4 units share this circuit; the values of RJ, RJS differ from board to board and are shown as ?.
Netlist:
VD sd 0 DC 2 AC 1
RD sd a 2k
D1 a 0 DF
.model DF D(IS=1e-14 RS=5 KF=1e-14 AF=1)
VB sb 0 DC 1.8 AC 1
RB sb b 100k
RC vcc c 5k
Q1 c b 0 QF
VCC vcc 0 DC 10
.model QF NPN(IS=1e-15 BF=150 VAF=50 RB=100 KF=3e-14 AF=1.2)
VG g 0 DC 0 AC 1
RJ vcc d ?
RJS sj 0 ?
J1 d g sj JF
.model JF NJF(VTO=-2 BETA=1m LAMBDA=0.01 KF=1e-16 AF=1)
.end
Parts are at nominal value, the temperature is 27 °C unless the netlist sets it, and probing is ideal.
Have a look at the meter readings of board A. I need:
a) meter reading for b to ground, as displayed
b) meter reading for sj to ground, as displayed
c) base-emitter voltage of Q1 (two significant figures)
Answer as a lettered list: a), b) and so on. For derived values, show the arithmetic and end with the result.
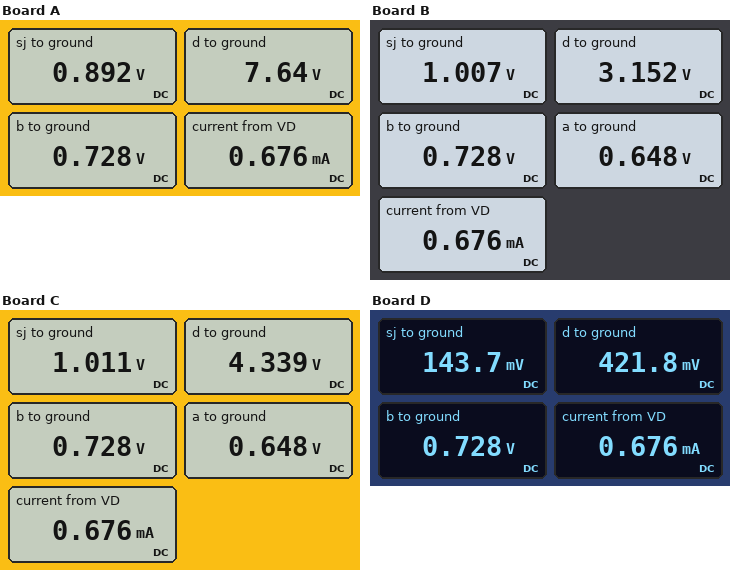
a) 0.728 V
b) 0.892 V
c) 728 mV = 730 mV
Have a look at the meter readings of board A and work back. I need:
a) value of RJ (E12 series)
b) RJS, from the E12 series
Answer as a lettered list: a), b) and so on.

a) 1.8 kΩ
b) 680 Ω
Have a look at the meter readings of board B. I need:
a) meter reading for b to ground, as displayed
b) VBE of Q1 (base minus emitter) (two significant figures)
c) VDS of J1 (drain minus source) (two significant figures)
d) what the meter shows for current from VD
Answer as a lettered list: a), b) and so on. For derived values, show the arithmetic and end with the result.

a) 0.728 V
b) 728 mV = 730 mV
c) 3.152 V - 1.007 V = 2.1 V
d) 0.676 mA
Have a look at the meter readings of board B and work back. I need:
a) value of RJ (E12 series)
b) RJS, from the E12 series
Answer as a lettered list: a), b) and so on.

a) 6.8 kΩ
b) 1 kΩ
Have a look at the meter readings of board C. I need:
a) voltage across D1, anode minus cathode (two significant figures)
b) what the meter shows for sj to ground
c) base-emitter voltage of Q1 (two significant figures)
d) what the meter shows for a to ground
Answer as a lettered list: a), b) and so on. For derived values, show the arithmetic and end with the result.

a) 648 mV = 650 mV
b) 1.011 V
c) 728 mV = 730 mV
d) 0.648 V
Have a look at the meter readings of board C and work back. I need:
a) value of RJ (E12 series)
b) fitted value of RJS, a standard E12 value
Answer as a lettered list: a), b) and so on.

a) 5.6 kΩ
b) 1 kΩ
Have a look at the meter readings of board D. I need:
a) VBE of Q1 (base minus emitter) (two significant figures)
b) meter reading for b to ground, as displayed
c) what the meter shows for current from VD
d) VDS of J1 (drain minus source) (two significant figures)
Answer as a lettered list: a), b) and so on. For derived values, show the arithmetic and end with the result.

a) 728 mV = 730 mV
b) 0.728 V
c) 0.676 mA
d) 421.8 mV - 143.7 mV = 280 mV
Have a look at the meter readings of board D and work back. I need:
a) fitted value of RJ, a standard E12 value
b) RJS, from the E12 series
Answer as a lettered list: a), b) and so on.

a) 10 kΩ
b) 150 Ω
